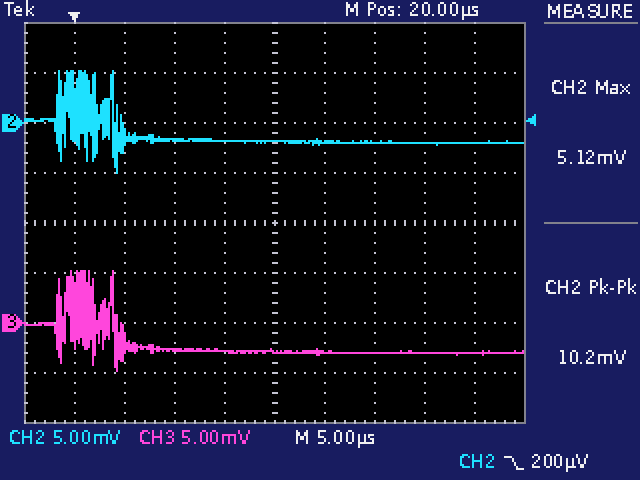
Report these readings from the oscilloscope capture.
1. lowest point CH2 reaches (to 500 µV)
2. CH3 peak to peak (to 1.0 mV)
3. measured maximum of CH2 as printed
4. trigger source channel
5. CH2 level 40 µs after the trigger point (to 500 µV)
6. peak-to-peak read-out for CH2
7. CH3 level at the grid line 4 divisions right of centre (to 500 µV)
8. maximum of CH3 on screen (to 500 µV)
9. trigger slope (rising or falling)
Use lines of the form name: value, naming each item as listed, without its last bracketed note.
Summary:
lowest point CH2 reaches: -5.0 mV
CH3 peak to peak: 10.0 mV
measured maximum of CH2 as printed: 5.12 mV
trigger source channel: CH2
CH2 level 40 µs after the trigger point: -2.0 mV
peak-to-peak read-out for CH2: 10.2 mV
CH3 level at the grid line 4 divisions right of centre: -3.0 mV
maximum of CH3 on screen: 5.0 mV
trigger slope: falling
